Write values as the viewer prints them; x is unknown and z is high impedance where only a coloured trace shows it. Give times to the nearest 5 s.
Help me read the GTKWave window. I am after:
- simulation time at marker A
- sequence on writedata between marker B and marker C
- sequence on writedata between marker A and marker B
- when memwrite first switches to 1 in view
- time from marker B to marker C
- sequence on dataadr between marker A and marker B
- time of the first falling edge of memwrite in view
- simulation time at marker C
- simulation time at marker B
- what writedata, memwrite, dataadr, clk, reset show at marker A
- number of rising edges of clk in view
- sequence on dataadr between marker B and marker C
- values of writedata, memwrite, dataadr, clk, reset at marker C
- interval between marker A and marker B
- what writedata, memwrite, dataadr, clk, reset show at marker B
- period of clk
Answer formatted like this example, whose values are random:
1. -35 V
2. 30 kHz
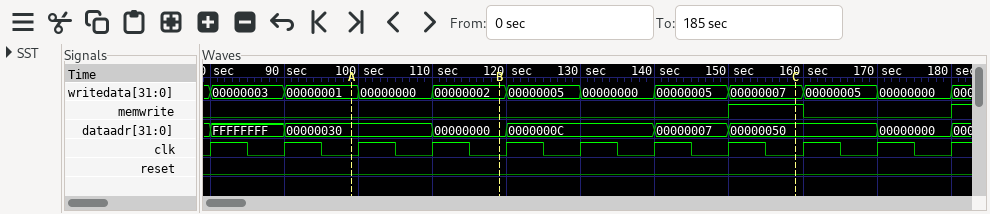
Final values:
1. 100 s
2. 00000002, 00000005, 00000000, 00000005, 00000007
3. 00000001, 00000000, 00000002
4. 150 s
5. 40 s
6. 00000030, 00000000
7. 160 s
8. 160 s
9. 120 s
10. writedata=00000001, memwrite=0, dataadr=00000030, clk=0, reset=0
11. 11
12. 00000000, 0000000C, 00000007, 00000050
13. writedata=00000007, memwrite=1, dataadr=00000050, clk=0, reset=0
14. 20 s
15. writedata=00000002, memwrite=0, dataadr=00000000, clk=0, reset=0
16. 10 s
